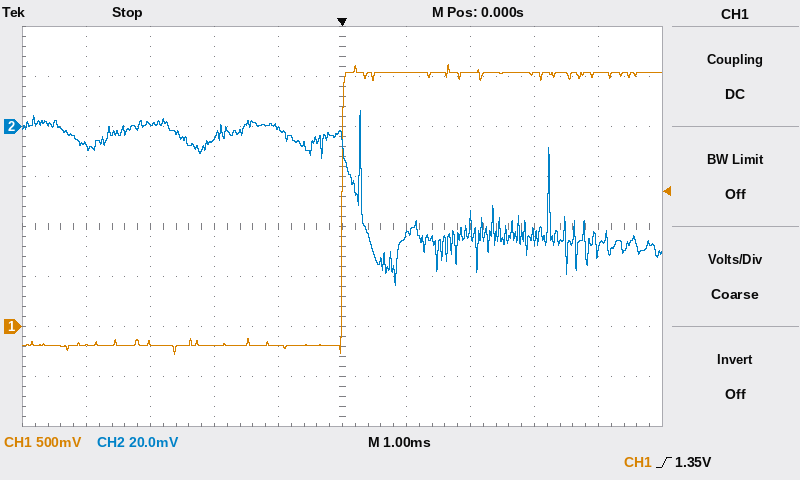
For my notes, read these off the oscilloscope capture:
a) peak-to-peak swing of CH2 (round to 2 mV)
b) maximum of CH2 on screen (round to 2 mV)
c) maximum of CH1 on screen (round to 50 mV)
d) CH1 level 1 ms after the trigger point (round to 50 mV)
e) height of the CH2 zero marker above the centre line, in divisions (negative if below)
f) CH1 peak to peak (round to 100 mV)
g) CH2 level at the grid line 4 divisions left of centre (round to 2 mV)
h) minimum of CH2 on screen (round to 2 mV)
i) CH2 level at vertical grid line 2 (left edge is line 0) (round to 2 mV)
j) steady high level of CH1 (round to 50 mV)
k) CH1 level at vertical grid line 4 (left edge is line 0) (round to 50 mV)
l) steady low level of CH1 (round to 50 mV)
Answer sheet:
70 mV
6 mV
2.60 V
2.55 V
+2.0 div
2.90 V
-8 mV
-64 mV
2 mV
2.55 V
-200 mV
-200 mV
